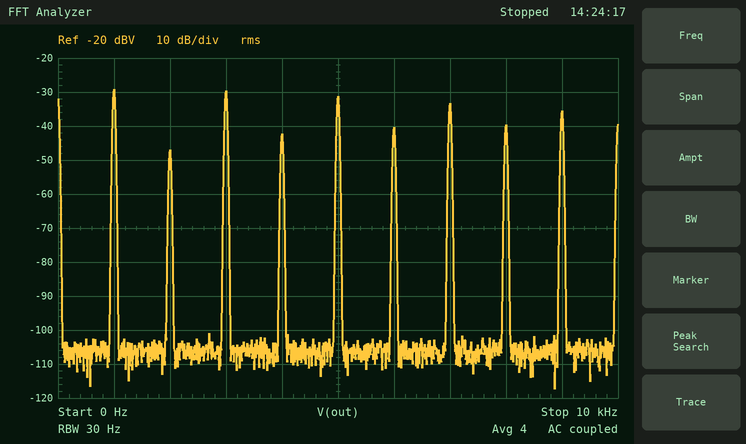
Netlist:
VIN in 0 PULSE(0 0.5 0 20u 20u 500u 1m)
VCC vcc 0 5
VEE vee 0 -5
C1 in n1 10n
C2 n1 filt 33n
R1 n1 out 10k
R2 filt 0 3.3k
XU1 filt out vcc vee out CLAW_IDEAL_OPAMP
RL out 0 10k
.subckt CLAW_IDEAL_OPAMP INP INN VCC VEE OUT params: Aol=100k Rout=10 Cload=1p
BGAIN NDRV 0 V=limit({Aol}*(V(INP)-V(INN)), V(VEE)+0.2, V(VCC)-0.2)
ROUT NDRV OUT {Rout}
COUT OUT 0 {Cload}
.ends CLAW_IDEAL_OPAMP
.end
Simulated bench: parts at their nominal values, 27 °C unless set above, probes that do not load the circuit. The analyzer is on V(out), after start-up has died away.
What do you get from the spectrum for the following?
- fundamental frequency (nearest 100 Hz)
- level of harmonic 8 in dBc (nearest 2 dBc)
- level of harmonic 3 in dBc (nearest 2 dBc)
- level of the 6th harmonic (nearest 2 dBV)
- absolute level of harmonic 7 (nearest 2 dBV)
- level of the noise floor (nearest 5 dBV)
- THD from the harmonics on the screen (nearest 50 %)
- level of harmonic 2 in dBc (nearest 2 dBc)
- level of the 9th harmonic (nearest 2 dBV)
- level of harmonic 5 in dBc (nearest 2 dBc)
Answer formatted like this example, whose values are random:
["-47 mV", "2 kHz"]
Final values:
["1.0 kHz", "-10 dBc", "0 dBc", "-40 dBV", "-34 dBV", "-105 dBV", "150 %", "-18 dBc", "-36 dBV", "-2 dBc"]
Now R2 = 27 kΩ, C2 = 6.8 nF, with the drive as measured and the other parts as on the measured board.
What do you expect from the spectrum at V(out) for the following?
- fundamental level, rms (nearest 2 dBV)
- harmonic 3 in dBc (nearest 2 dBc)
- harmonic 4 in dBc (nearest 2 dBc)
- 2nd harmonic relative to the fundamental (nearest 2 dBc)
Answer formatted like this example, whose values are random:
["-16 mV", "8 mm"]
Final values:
["-16 dBV", "-6 dBc", "-20 dBc", "-20 dBc"]
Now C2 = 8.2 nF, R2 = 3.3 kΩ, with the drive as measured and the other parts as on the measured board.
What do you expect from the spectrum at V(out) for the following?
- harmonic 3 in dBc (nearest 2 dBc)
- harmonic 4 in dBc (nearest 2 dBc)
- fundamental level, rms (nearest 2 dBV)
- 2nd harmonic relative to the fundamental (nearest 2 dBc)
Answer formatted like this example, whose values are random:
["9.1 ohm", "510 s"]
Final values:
["2 dBc", "-10 dBc", "-36 dBV", "-16 dBc"]
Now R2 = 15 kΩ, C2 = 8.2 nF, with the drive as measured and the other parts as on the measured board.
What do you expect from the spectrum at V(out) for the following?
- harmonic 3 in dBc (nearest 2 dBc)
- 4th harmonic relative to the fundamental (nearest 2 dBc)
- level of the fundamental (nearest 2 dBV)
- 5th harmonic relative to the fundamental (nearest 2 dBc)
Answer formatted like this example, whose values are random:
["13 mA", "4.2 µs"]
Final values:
["-2 dBc", "-16 dBc", "-22 dBV", "-6 dBc"]
